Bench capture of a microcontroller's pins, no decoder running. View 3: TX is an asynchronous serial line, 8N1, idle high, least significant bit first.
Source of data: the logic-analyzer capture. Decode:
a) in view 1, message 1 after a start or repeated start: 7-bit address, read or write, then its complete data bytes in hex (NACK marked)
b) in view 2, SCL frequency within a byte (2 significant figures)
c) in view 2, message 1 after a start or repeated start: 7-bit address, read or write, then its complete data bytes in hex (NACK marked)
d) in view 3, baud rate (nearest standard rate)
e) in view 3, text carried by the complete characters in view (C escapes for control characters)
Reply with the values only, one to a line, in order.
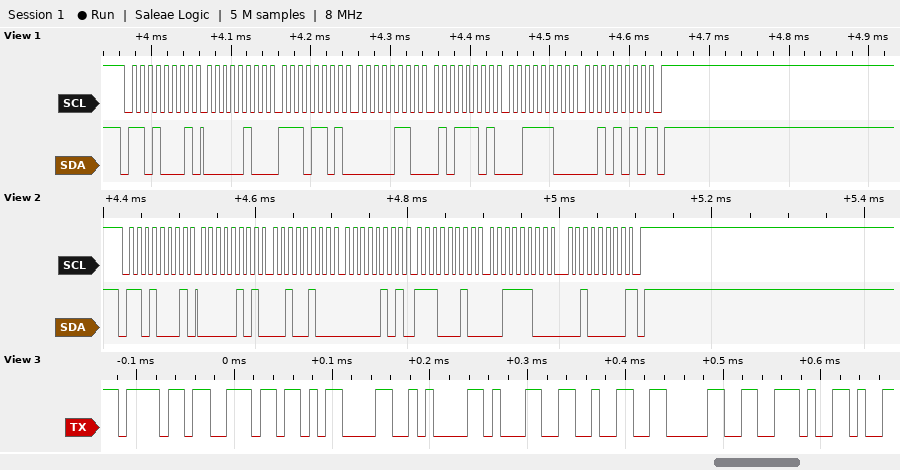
0x68 read: 04 ED 06 5D 3C 2A NACK
100 kHz
0x68 read: 05 24 05 E2 3C 20 NACK
115200 baud
"on\r\n120."
